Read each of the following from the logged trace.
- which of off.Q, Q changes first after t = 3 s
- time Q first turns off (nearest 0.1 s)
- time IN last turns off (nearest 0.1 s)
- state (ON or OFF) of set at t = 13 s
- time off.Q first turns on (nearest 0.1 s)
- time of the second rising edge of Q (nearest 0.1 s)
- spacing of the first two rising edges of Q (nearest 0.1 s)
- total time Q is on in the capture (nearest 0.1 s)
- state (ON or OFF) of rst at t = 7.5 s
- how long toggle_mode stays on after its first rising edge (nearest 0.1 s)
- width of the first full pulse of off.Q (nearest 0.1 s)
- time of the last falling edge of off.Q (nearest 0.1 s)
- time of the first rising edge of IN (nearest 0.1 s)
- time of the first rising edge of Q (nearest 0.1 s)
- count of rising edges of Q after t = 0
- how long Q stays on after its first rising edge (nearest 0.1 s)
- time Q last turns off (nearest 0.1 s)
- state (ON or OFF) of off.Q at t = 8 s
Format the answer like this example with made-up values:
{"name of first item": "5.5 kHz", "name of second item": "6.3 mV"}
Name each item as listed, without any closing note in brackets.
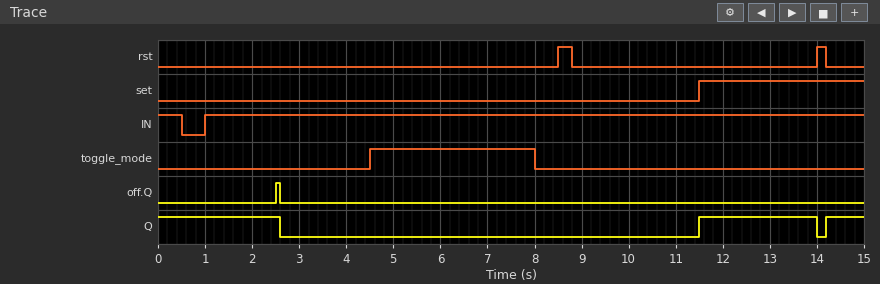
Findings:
{"which of off.Q, Q changes first after t = 3 s": "Q", "time Q first turns off": "2.6 s", "time IN last turns off": "0.5 s", "state (ON or OFF) of set at t = 13 s": "ON", "time off.Q first turns on": "2.5 s", "time of the second rising edge of Q": "14.2 s", "spacing of the first two rising edges of Q": "2.7 s", "total time Q is on in the capture": "5.9 s", "state (ON or OFF) of rst at t = 7.5 s": "OFF", "how long toggle_mode stays on after its first rising edge": "3.5 s", "width of the first full pulse of off.Q": "0.1 s", "time of the last falling edge of off.Q": "2.6 s", "time of the first rising edge of IN": "1.0 s", "time of the first rising edge of Q": "11.5 s", "count of rising edges of Q after t = 0": "2", "how long Q stays on after its first rising edge": "2.5 s", "time Q last turns off": "14.0 s", "state (ON or OFF) of off.Q at t = 8 s": "OFF"}
